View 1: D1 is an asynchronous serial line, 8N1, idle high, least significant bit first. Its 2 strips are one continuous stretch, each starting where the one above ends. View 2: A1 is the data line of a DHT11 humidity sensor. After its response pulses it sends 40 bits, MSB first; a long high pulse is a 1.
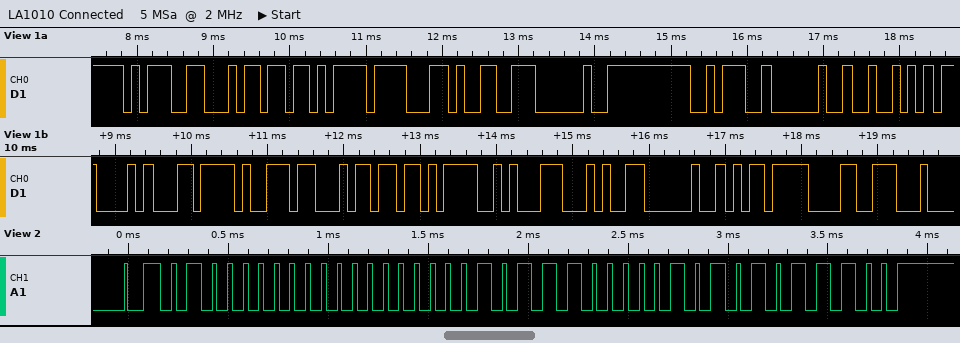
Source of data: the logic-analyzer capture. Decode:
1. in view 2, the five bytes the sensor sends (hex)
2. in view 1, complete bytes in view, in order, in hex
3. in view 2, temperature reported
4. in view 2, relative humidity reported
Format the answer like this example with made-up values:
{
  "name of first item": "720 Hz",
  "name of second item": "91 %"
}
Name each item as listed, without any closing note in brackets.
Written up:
{
  "in view 2, the five bytes the sensor sends": "40 00 17 05 5C",
  "in view 1, complete bytes in view, in order, in hex": "9D B4 EB 8F 99 20 3A 20 52 43 EC B9 B4 EB 8A 94 20 ED 98",
  "in view 2, temperature reported": "23.5 °C",
  "in view 2, relative humidity reported": "64 %"
}
